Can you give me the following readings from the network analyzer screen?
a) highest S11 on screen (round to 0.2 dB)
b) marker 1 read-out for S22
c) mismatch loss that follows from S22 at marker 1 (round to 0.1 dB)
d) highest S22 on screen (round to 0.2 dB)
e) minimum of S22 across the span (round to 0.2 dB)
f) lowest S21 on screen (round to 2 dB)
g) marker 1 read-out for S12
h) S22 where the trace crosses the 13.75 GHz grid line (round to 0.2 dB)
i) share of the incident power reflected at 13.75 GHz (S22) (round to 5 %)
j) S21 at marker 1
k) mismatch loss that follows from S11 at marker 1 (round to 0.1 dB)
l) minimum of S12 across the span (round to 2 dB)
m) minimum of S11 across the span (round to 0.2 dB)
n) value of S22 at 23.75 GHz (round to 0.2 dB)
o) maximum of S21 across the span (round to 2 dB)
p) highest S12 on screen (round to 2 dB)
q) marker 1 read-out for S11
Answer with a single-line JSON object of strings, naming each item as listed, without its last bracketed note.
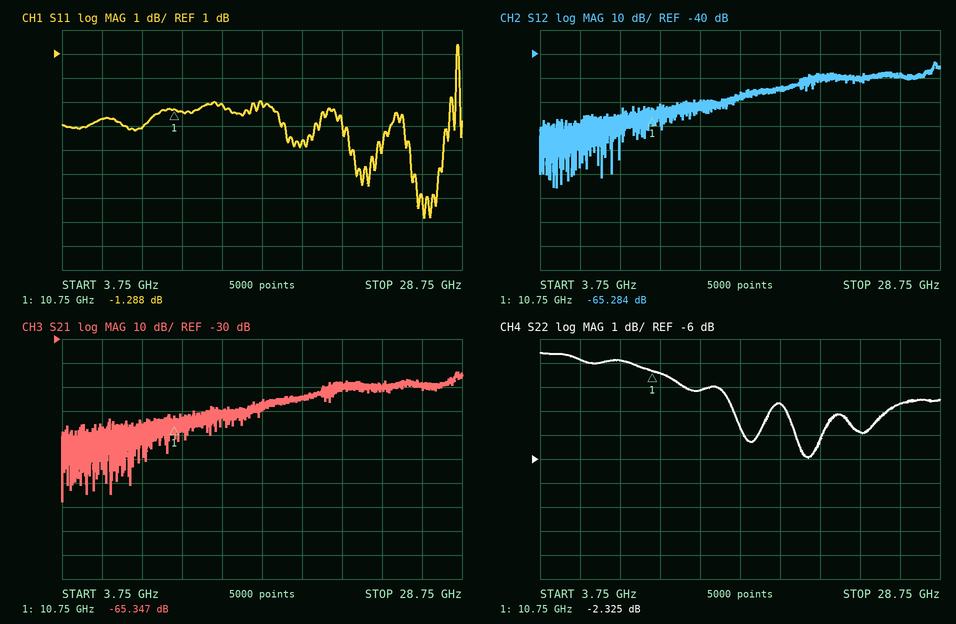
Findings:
{"highest S11 on screen": "1.4 dB", "marker 1 read-out for S22": "-2.325 dB", "mismatch loss that follows from S22 at marker 1": "3.8 dB", "highest S22 on screen": "-1.6 dB", "minimum of S22 across the span": "-6.0 dB", "lowest S21 on screen": "-98 dB", "marker 1 read-out for S12": "-65.284 dB", "S22 where the trace crosses the 13.75 GHz grid line": "-3.2 dB", "share of the incident power reflected at 13.75 GHz (S22)": "50 %", "S21 at marker 1": "-65.347 dB", "mismatch loss that follows from S11 at marker 1": "5.9 dB", "minimum of S12 across the span": "-96 dB", "minimum of S11 across the span": "-5.8 dB", "value of S22 at 23.75 GHz": "-4.8 dB", "maximum of S21 across the span": "-44 dB", "highest S12 on screen": "-44 dB", "marker 1 read-out for S11": "-1.288 dB"}
